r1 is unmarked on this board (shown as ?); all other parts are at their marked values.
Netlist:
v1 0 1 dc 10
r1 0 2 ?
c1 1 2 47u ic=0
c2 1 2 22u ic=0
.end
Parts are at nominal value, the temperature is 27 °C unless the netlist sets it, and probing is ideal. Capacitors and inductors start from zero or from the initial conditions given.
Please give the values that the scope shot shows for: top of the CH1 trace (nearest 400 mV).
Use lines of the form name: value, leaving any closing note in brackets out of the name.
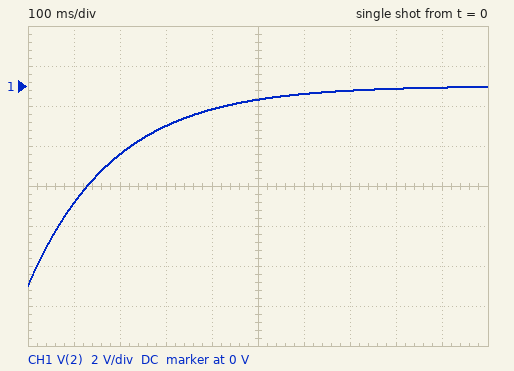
top of the CH1 trace: 0 V
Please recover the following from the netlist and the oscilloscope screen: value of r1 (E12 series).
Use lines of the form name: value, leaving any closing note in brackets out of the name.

value of r1: 2.7 kΩ
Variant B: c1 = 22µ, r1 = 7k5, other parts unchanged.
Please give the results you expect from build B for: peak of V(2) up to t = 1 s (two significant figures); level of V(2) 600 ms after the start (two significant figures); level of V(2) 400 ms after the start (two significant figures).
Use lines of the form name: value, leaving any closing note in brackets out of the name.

peak of V(2) up to t = 1 s: -480 mV
level of V(2) 600 ms after the start: -1.6 V
level of V(2) 400 ms after the start: -3.0 V
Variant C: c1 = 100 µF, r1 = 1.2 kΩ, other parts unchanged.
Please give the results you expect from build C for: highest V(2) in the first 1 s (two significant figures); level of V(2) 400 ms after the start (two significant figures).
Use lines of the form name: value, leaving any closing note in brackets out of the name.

highest V(2) in the first 1 s: -11 mV
level of V(2) 400 ms after the start: -650 mV
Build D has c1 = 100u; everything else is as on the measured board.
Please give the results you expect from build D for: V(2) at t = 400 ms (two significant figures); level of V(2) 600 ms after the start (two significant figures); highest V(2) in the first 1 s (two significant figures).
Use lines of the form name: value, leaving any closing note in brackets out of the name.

V(2) at t = 400 ms: -3.0 V
level of V(2) 600 ms after the start: -1.6 V
highest V(2) in the first 1 s: -480 mV
